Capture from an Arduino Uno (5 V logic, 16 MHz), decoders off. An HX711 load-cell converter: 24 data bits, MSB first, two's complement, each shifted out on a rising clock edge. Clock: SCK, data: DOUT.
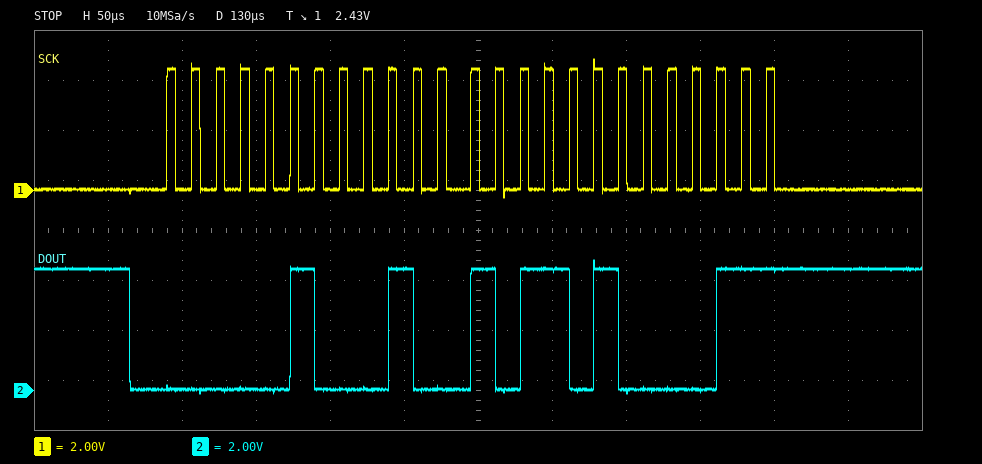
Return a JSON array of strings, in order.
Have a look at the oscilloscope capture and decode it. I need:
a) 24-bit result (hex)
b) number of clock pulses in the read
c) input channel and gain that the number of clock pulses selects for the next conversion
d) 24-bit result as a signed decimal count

["0x044B43", "25", "channel A, gain 128", "281411"]
